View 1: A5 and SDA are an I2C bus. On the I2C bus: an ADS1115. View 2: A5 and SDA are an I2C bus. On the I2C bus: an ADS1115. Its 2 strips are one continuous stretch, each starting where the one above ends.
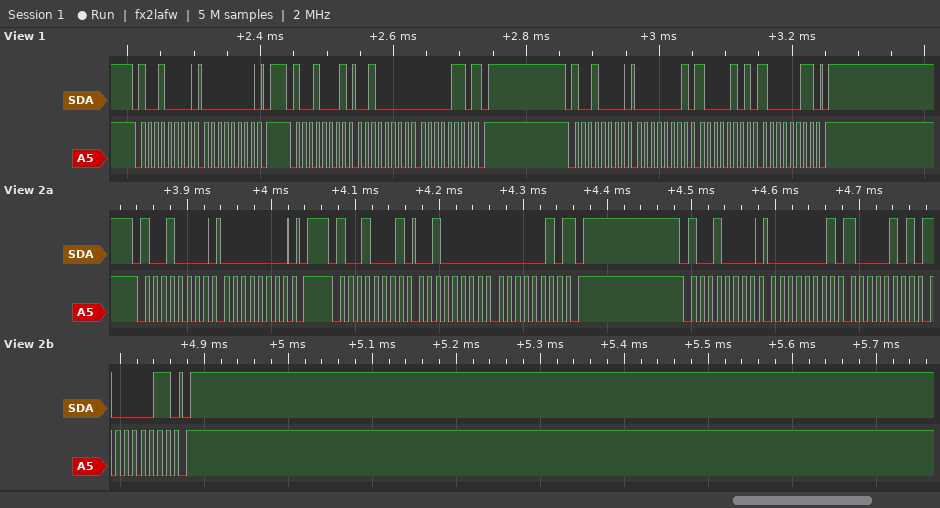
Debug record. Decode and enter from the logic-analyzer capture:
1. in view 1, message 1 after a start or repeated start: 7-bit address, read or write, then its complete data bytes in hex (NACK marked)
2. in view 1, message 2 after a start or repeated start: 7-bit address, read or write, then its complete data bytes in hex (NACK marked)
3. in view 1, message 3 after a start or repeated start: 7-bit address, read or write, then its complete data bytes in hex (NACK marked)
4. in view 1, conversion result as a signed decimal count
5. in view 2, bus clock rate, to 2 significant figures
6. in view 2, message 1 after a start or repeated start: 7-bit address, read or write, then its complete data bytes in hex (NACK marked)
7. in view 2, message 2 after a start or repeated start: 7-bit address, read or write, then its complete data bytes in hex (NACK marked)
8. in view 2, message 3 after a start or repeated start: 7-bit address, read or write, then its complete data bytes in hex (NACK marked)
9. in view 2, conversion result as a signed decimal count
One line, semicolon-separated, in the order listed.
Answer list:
0x48 write: 00; 0x48 read: 20 06 NACK; 0x48 write: 01 85 83; 8198; 100 kHz; 0x48 write: 00; 0x48 read: 20 02 NACK; 0x48 write: 01 85 83; 8194
